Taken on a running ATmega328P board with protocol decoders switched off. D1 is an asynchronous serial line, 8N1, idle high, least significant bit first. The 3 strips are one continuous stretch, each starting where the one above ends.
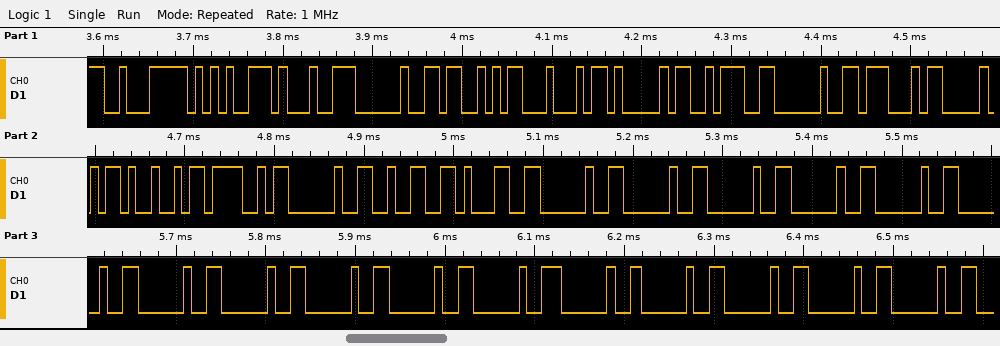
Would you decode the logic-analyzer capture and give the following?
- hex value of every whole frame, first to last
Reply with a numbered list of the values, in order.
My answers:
1. E2 95 91 20 53 44 41 3A 20 47 50 49 4F 20 32 31 20 20 20 20 20 20 20 20 20 20 20 20 20 20 20 20
